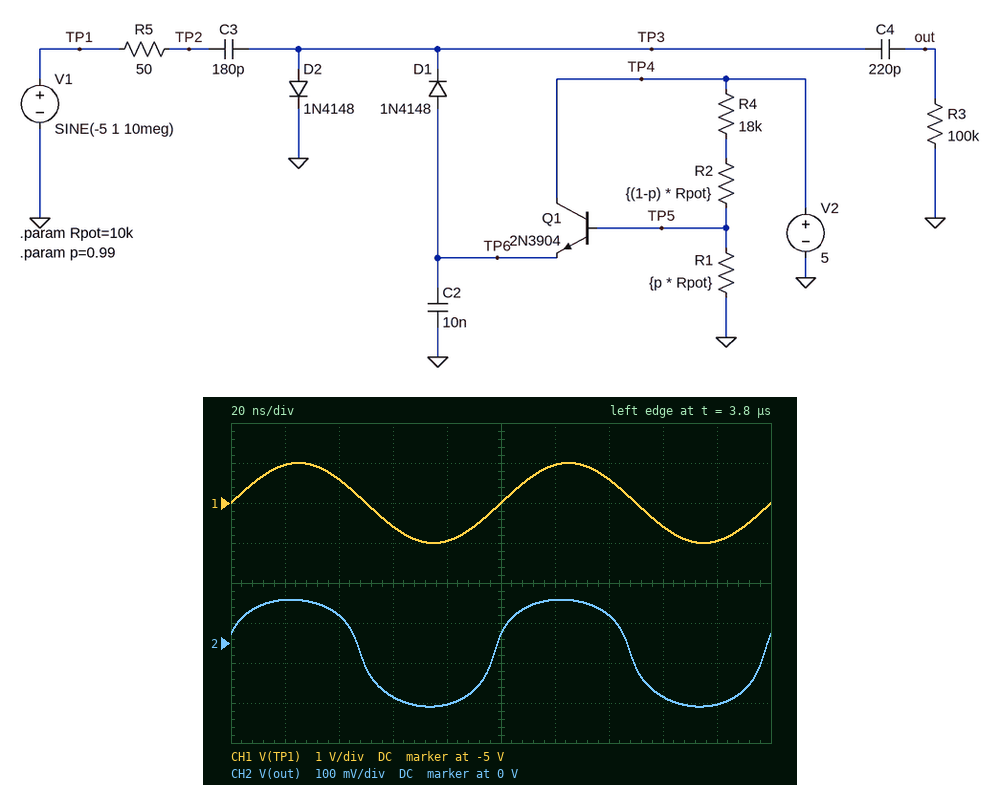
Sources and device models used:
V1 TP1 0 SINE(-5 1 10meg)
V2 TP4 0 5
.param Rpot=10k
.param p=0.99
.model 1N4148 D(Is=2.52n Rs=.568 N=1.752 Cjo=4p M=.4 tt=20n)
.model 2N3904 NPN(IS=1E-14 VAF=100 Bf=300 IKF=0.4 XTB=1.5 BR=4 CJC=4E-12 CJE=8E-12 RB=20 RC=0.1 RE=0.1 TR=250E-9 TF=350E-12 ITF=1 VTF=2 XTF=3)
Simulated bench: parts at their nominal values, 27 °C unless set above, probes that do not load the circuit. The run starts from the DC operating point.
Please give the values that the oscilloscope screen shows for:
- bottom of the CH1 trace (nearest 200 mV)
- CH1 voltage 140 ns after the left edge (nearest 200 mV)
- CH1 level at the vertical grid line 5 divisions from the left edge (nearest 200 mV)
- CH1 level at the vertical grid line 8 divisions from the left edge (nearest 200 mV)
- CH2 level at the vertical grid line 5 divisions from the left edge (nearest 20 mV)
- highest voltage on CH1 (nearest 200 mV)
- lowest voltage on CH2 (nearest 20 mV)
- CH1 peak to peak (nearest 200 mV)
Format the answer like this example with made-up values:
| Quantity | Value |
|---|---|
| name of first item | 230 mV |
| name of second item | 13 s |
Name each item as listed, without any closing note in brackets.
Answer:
| Quantity | Value |
|---|---|
| bottom of the CH1 trace | -6.0 V |
| CH1 voltage 140 ns after the left edge | -4.4 V |
| CH1 level at the vertical grid line 5 divisions from the left edge | -5.0 V |
| CH1 level at the vertical grid line 8 divisions from the left edge | -5.6 V |
| CH2 level at the vertical grid line 5 divisions from the left edge | 20 mV |
| highest voltage on CH1 | -4.0 V |
| lowest voltage on CH2 | -160 mV |
| CH1 peak to peak | 2.0 V |
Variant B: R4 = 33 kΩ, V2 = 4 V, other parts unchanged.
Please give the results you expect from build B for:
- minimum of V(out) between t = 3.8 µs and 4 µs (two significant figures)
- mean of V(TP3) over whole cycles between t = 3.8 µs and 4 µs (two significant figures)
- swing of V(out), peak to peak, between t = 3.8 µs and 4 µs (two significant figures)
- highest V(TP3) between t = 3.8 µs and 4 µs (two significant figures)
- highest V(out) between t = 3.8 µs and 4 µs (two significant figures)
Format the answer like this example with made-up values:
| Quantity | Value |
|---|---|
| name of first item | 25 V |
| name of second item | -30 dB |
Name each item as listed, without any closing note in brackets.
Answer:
| Quantity | Value |
|---|---|
| minimum of V(out) between t = 3.8 µs and 4 µs | -600 mV |
| mean of V(TP3) over whole cycles between t = 3.8 µs and 4 µs | 130 mV |
| swing of V(out), peak to peak, between t = 3.8 µs and 4 µs | 1.0 V |
| highest V(TP3) between t = 3.8 µs and 4 µs | 630 mV |
| highest V(out) between t = 3.8 µs and 4 µs | 410 mV |
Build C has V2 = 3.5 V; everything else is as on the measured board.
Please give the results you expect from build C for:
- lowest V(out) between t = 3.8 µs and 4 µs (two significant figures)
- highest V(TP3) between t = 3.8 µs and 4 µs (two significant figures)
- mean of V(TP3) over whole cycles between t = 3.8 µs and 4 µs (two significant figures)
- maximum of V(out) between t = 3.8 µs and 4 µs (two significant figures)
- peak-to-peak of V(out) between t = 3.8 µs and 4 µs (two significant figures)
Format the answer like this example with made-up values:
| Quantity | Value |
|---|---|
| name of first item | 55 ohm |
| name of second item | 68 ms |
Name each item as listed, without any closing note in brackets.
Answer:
| Quantity | Value |
|---|---|
| lowest V(out) between t = 3.8 µs and 4 µs | -440 mV |
| highest V(TP3) between t = 3.8 µs and 4 µs | 650 mV |
| mean of V(TP3) over whole cycles between t = 3.8 µs and 4 µs | 280 mV |
| maximum of V(out) between t = 3.8 µs and 4 µs | 300 mV |
| peak-to-peak of V(out) between t = 3.8 µs and 4 µs | 740 mV |
